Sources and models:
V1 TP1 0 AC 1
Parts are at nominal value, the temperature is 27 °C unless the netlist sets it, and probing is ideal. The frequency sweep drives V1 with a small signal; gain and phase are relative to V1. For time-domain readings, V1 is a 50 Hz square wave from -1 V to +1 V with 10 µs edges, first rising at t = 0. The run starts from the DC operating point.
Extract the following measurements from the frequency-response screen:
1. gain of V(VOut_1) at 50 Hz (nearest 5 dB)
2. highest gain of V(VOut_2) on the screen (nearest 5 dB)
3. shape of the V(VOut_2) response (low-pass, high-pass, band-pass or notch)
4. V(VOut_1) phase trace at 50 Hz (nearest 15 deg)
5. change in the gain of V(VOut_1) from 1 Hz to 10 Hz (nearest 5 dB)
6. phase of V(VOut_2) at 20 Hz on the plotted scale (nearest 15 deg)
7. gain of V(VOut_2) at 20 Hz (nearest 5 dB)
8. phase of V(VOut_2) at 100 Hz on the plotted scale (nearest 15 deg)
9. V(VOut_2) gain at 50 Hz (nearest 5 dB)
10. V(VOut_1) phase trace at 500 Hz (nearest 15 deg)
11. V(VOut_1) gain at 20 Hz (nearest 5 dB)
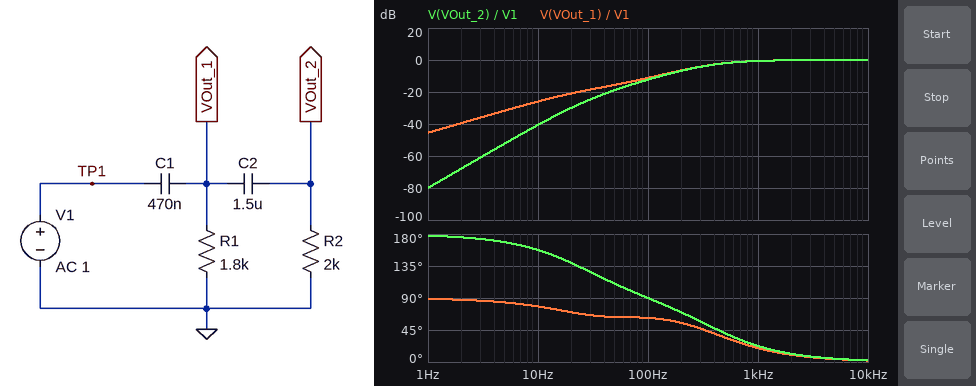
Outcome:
-15 dB
0 dB
high-pass
60 deg
20 dB
135 deg
-30 dB
90 deg
-20 dB
30 deg
-20 dB
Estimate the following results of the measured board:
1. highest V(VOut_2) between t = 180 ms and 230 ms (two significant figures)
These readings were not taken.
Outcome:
2.0 V
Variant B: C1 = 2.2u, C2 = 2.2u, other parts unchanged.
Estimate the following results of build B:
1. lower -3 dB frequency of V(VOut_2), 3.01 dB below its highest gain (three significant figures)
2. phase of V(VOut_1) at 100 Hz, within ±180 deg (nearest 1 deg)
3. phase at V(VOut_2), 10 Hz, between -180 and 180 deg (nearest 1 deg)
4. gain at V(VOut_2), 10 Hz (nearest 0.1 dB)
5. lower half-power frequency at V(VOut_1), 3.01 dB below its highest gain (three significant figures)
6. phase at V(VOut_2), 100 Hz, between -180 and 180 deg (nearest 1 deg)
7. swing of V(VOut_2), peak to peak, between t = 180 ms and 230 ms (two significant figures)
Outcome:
99.8 Hz
33 deg
140 deg
-24.9 dB
86.2 Hz
53 deg
4.2 V
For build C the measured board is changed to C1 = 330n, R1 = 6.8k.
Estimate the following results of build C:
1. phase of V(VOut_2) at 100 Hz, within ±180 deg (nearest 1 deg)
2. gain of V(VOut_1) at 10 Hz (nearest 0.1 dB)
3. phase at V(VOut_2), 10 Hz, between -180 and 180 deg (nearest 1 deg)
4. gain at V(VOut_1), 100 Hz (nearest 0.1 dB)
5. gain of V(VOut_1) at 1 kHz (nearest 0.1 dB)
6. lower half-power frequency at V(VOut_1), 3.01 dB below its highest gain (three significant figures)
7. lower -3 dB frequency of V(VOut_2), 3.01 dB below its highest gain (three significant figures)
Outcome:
80 deg
-19.6 dB
135 deg
-10.3 dB
-0.5 dB
347 Hz
355 Hz
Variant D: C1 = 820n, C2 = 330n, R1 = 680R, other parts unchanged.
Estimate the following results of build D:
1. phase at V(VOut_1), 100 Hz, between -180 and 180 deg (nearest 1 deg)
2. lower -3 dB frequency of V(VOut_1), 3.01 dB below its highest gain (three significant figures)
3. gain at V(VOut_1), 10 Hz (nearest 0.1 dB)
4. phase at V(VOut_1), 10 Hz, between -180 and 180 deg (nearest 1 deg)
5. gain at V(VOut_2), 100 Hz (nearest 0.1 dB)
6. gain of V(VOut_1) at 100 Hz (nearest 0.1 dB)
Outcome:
66 deg
405 Hz
-29.1 dB
87 deg
-18.7 dB
-10.3 dB
